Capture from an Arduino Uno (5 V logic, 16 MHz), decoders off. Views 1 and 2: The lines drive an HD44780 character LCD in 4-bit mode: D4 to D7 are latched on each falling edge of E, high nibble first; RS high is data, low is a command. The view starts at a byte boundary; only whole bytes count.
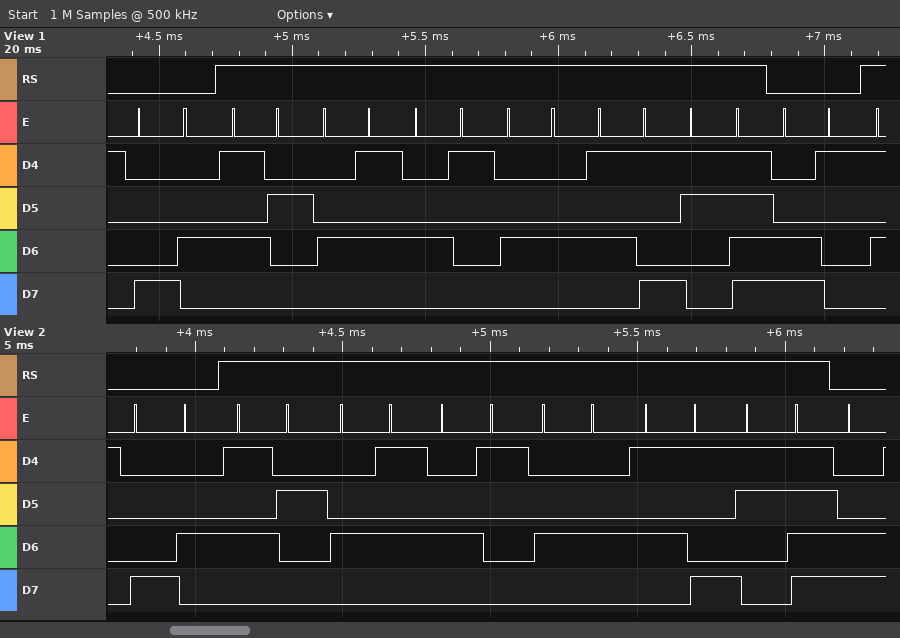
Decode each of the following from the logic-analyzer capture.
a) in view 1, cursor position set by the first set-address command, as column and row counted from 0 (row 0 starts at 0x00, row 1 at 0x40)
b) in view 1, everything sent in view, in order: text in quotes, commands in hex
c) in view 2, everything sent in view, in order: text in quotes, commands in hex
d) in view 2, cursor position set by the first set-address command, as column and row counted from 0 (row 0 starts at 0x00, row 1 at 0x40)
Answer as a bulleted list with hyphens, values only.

- column 4, row 0
- 0x84 "READY?" 0xC1
- 0x84 "READY?"
- column 4, row 0
